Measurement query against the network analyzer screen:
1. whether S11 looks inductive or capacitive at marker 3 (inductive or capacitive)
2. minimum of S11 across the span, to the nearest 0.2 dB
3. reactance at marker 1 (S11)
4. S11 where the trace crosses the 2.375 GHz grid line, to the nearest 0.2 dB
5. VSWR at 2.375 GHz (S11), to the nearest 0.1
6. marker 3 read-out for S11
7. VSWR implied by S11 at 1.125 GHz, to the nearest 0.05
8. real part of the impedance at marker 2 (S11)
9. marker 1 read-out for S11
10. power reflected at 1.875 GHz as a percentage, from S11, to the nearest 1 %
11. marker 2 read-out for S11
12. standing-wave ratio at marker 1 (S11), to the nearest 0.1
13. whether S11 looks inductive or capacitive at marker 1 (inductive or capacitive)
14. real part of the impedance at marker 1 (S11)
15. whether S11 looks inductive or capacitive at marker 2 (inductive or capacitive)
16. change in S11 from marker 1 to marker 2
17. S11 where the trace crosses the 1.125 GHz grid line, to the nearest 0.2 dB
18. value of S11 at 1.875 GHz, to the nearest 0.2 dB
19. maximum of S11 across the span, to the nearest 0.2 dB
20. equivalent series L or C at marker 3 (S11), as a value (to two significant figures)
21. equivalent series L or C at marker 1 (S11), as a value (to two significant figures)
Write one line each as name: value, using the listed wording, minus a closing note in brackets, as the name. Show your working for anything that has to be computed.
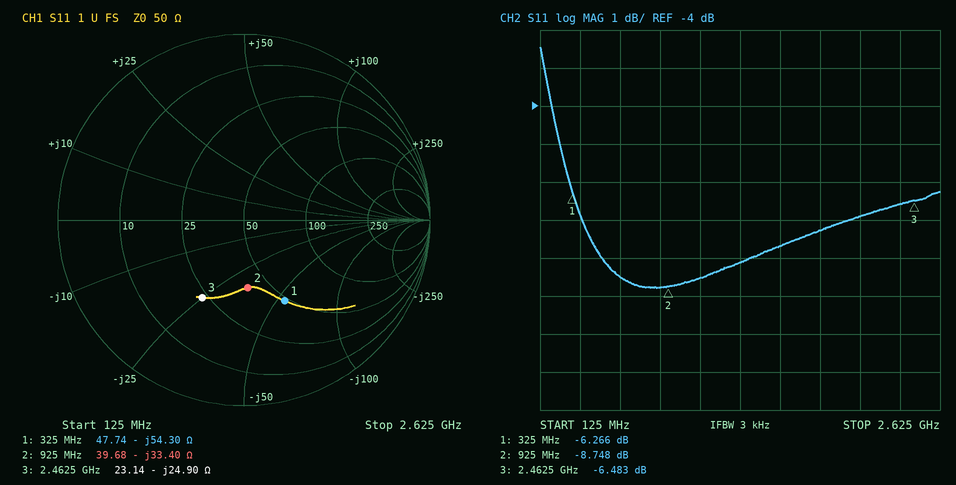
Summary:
whether S11 looks inductive or capacitive at marker 3: capacitive
minimum of S11 across the span, to the nearest 0.2 dB: -8.8 dB
reactance at marker 1: -54.30 Ω
S11 where the trace crosses the 2.375 GHz grid line, to the nearest 0.2 dB: -6.6 dB
VSWR at 2.375 GHz (S11), to the nearest 0.1: |Γ| = 10^(-6.6/20) = 0.4677; VSWR = (1 + 0.4677)/(1 − 0.4677) ≈ 2.8
marker 3 read-out for S11: -6.483 dB
VSWR implied by S11 at 1.125 GHz, to the nearest 0.05: |Γ| = 10^(-8.6/20) = 0.3715; VSWR = (1 + 0.3715)/(1 − 0.3715) ≈ 2.18, so 2.20 to the nearest 0.05
real part of the impedance at marker 2: 39.68 Ω
marker 1 read-out for S11: -6.266 dB
power reflected at 1.875 GHz as a percentage, from S11, to the nearest 1 %: 10^(-7.2/10) ≈ 19 %
marker 2 read-out for S11: -8.748 dB
standing-wave ratio at marker 1 (S11), to the nearest 0.1: 2.9
whether S11 looks inductive or capacitive at marker 1: capacitive
real part of the impedance at marker 1: 47.74 Ω
whether S11 looks inductive or capacitive at marker 2: capacitive
change in S11 from marker 1 to marker 2: -8.748 − (-6.266) = -2.482 dB
S11 where the trace crosses the 1.125 GHz grid line, to the nearest 0.2 dB: -8.6 dB
value of S11 at 1.875 GHz, to the nearest 0.2 dB: -7.2 dB
maximum of S11 across the span, to the nearest 0.2 dB: -2.4 dB
equivalent series L or C at marker 3 (S11), as a value: C = 1/(2π × 2.4625 GHz × 24.9 Ω) ≈ 2.6 pF
equivalent series L or C at marker 1 (S11), as a value: C = 1/(2π × 325 MHz × 54.3 Ω) ≈ 9.0 pF
